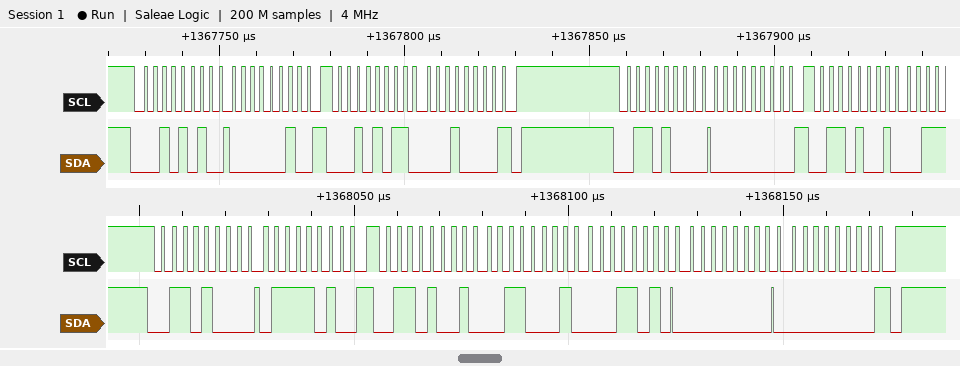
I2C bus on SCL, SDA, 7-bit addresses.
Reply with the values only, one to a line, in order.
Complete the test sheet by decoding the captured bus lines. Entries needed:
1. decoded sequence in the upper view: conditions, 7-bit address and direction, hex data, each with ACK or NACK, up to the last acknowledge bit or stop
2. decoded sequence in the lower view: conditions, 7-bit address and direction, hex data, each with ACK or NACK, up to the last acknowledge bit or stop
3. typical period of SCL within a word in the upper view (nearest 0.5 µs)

start, address 15 write ACK, 02 ACK, repeated start, address 15 read ACK, 10 NACK, stop, start, address 34 write ACK, 00 ACK, repeated start, address 34 read ACK
start, address 34 write ACK, 7A ACK, repeated start, address 34 read ACK, 31 ACK, 1A ACK, 00 ACK, 00 NACK, stop
2.5 µs
